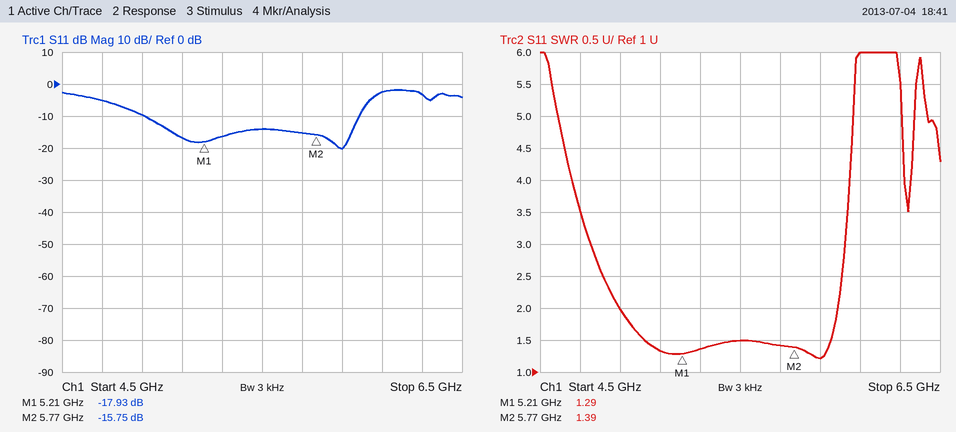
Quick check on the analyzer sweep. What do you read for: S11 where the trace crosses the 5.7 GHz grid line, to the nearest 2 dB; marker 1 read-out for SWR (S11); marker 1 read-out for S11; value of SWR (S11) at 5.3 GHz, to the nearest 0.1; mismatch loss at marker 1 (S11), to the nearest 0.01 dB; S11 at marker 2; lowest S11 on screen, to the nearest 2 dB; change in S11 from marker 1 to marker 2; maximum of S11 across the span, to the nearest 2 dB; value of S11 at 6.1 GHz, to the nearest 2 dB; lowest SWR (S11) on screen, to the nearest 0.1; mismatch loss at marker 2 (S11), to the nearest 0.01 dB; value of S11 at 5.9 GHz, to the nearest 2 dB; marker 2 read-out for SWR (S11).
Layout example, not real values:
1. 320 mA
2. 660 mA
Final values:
1. -16 dB
2. 1.29
3. -17.93 dB
4. 1.4
5. 0.07 dB
6. -15.75 dB
7. -20 dB
8. 2.18 dB
9. -2 dB
10. -2 dB
11. 1.2
12. 0.12 dB
13. -20 dB
14. 1.39
